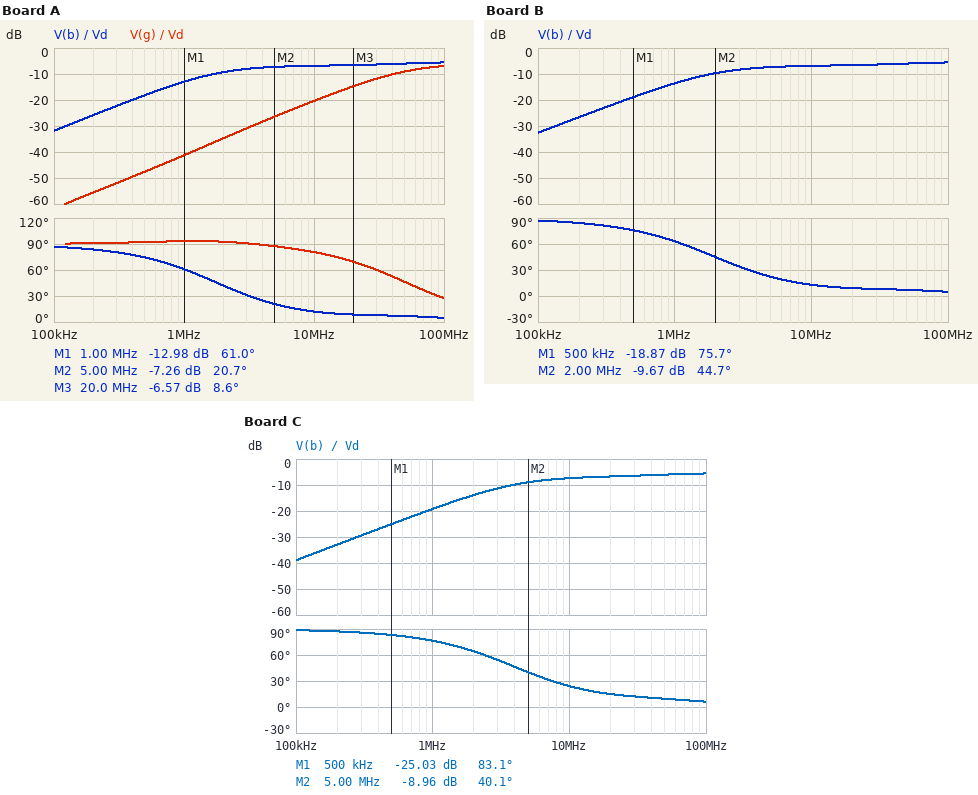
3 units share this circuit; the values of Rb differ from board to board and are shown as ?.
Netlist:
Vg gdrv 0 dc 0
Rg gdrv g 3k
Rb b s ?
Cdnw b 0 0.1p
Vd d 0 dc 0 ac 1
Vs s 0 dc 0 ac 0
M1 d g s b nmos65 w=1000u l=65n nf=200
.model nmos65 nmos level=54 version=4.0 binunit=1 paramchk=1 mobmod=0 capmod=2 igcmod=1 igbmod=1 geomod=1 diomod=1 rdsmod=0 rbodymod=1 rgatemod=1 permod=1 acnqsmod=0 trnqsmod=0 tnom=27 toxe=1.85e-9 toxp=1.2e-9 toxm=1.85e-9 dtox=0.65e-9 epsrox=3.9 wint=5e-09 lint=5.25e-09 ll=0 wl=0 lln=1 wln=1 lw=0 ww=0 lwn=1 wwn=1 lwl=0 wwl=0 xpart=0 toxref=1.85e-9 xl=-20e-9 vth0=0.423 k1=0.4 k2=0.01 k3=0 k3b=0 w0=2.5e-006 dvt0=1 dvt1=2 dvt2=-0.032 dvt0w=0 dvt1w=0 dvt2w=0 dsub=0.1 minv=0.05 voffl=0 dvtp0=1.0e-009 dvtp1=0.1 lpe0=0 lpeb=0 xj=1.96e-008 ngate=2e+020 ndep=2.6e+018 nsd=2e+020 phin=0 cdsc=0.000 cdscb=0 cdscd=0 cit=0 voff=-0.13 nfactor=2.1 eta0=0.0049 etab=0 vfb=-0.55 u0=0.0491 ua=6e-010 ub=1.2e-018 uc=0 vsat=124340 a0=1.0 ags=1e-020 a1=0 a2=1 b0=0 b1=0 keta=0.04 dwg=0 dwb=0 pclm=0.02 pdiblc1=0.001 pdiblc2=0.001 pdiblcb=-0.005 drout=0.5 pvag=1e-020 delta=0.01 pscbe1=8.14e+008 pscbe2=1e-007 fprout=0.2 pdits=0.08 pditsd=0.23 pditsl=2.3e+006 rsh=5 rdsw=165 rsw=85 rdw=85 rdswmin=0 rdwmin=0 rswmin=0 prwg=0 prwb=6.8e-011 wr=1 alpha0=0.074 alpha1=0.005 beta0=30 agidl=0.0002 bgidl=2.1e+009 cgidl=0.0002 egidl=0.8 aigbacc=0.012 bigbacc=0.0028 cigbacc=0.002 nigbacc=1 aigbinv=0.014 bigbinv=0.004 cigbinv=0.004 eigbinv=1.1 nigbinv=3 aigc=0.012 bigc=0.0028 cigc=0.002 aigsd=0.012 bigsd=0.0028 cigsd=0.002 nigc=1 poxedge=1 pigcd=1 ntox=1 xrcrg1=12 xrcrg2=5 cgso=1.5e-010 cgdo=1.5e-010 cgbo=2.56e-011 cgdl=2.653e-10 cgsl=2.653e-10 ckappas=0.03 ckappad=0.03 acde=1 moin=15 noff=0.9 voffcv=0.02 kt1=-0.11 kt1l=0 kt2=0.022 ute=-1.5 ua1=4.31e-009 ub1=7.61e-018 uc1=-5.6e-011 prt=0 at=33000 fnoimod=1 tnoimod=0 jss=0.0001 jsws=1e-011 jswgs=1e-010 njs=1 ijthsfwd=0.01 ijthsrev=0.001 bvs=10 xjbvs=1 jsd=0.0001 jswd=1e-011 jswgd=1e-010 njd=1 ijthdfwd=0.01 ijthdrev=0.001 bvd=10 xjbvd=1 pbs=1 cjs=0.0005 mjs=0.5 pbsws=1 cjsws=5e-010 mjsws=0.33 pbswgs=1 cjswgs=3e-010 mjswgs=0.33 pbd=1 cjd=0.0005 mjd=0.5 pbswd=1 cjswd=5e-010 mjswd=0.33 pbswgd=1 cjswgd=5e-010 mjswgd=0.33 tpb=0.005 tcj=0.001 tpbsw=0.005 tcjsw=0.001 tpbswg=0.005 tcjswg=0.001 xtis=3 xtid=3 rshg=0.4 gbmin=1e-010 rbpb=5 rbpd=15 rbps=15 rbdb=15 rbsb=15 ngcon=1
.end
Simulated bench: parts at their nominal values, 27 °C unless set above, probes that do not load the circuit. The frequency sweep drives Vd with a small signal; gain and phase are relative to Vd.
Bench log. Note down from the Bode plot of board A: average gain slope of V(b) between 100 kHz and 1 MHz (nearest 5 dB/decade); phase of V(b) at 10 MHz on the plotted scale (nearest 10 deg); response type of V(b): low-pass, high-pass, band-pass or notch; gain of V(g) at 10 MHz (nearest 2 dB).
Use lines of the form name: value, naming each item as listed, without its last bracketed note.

average gain slope of V(b) between 100 kHz and 1 MHz: 20 dB/decade
phase of V(b) at 10 MHz on the plotted scale: 10 deg
response type of V(b): low-pass, high-pass, band-pass or notch: high-pass
gain of V(g) at 10 MHz: -20 dB
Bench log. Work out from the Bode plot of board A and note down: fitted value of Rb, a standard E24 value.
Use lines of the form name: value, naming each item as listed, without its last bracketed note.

fitted value of Rb, a standard E24 value: 82 kΩ
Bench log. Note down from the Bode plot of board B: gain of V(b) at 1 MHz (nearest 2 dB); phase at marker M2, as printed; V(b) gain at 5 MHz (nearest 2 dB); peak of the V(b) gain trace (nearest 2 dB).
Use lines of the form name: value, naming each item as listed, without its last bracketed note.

gain of V(b) at 1 MHz: -14 dB
phase at marker M2, as printed: 44.7 deg
V(b) gain at 5 MHz: -8 dB
peak of the V(b) gain trace: -6 dB
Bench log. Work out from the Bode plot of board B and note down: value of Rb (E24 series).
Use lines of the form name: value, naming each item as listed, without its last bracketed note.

value of Rb: 75 kΩ
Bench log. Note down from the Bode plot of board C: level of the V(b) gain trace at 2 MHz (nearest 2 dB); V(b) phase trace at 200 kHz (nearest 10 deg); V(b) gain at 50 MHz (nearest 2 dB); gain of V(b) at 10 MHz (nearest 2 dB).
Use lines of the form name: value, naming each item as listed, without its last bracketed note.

level of the V(b) gain trace at 2 MHz: -14 dB
V(b) phase trace at 200 kHz: 90 deg
V(b) gain at 50 MHz: -6 dB
gain of V(b) at 10 MHz: -8 dB
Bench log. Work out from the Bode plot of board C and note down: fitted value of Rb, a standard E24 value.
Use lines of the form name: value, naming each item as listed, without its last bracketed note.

fitted value of Rb, a standard E24 value: 36 kΩ
